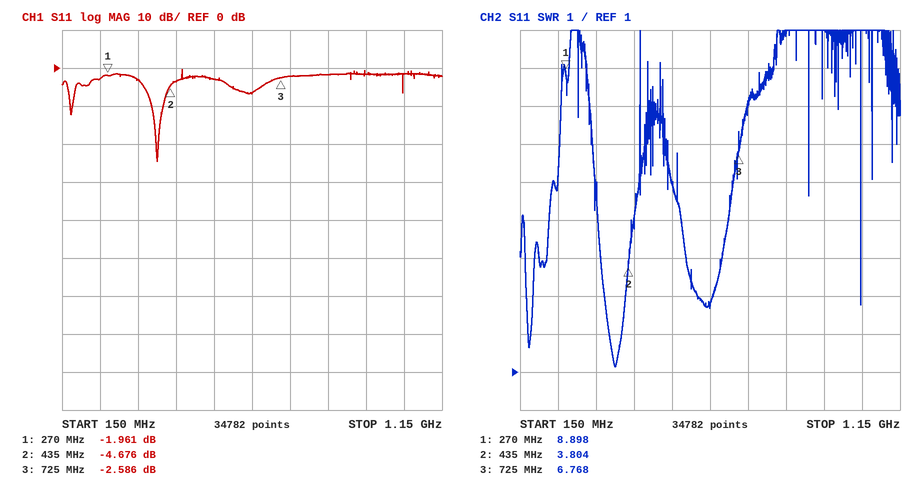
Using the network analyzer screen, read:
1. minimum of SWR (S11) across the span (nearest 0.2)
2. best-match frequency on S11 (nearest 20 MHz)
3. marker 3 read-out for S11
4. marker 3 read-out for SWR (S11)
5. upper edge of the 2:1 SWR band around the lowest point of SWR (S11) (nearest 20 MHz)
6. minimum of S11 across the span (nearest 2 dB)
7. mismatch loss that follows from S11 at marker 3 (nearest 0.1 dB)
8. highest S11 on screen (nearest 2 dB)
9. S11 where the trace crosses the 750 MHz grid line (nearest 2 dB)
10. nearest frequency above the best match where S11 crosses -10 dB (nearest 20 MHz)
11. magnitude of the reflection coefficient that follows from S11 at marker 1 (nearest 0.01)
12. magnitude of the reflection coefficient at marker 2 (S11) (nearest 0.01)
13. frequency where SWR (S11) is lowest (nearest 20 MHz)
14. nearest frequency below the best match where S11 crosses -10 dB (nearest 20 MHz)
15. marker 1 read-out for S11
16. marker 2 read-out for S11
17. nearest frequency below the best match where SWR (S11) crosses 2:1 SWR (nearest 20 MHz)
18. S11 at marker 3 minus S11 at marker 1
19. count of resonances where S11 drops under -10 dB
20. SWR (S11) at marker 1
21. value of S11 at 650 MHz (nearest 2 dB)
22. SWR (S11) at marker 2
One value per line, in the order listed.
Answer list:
1.2
400 MHz
-2.586 dB
6.768
420 MHz
-24 dB
3.5 dB
0 dB
-2 dB
420 MHz
0.80
0.58
400 MHz
380 MHz
-1.961 dB
-4.676 dB
380 MHz
-0.625 dB
2
8.898
-6 dB
3.804
